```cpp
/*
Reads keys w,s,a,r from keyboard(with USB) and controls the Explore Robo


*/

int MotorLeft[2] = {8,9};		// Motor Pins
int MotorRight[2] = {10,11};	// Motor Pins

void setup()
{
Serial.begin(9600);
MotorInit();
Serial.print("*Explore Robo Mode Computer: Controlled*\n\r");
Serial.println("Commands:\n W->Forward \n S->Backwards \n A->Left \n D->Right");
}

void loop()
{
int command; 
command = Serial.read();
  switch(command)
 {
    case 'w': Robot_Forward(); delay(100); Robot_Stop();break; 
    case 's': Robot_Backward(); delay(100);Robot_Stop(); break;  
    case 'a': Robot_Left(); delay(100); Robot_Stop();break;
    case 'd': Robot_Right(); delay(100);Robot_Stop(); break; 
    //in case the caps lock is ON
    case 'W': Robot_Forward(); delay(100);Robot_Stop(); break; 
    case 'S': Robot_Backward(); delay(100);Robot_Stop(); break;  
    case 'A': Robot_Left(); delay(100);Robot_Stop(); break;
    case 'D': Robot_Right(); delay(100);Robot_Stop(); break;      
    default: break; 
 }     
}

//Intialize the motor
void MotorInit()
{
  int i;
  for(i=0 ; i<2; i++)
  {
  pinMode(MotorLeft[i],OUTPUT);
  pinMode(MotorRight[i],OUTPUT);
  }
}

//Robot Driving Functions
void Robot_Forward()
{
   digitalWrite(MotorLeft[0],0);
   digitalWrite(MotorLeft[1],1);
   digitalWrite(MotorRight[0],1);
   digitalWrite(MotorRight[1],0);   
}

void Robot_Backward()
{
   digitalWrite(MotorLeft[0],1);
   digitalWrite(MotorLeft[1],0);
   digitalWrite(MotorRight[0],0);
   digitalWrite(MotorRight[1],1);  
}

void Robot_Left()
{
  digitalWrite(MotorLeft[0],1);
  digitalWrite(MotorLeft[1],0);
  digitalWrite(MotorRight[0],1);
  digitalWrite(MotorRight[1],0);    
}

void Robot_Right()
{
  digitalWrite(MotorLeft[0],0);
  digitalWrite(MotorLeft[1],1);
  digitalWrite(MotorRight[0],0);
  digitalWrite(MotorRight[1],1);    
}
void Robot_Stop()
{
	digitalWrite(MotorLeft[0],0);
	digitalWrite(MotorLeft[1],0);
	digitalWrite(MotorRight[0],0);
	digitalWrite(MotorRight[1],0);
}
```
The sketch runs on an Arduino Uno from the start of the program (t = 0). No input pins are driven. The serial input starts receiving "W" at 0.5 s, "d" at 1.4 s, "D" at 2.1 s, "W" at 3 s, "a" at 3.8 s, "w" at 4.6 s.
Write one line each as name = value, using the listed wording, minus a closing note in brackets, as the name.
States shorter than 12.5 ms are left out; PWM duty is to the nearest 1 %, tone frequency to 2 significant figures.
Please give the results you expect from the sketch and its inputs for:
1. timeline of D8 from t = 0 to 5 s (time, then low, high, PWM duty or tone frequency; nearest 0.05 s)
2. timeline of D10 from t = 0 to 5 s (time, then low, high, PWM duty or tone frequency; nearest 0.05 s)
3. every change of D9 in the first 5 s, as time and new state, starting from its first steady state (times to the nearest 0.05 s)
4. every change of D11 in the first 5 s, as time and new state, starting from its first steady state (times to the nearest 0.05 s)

timeline of D8 from t = 0 to 5 s = 0 s low; 3.8 s high; 3.9 s low
timeline of D10 from t = 0 to 5 s = 0 s low; 0.5 s high; 0.6 s low; 3 s high; 3.1 s low; 3.8 s high; 3.9 s low; 4.6 s high; 4.7 s low
every change of D9 in the first 5 s, as time and new state, starting from its first steady state = 0 s low; 0.5 s high; 0.6 s low; 1.4 s high; 1.5 s low; 2.1 s high; 2.2 s low; 3 s high; 3.1 s low; 4.6 s high; 4.7 s low
every change of D11 in the first 5 s, as time and new state, starting from its first steady state = 0 s low; 1.4 s high; 1.5 s low; 2.1 s high; 2.2 s low
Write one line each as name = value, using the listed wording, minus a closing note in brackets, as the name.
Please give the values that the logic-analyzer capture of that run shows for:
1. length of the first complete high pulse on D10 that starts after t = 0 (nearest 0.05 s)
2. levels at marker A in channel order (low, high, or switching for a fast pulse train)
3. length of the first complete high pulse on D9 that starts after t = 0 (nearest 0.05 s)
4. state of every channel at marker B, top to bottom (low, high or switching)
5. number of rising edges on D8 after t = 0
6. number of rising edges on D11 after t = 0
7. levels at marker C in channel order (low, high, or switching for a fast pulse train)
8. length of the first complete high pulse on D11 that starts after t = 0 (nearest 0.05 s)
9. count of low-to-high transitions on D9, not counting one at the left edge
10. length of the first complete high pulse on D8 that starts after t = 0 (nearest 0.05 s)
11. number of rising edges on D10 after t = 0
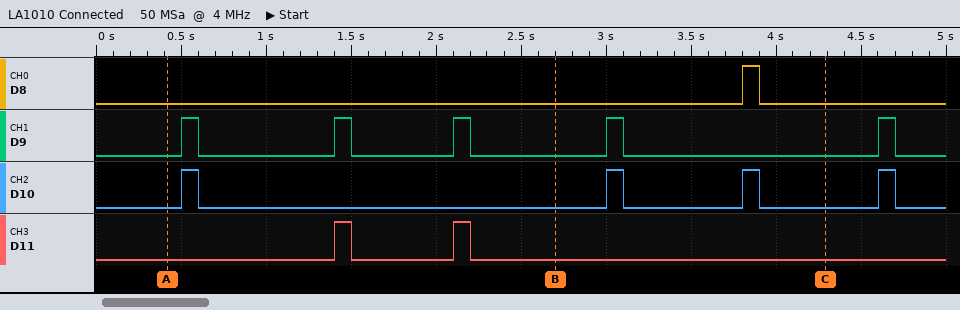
length of the first complete high pulse on D10 that starts after t = 0 = 0.10 s
levels at marker A in channel order = D8 low, D9 low, D10 low, D11 low
length of the first complete high pulse on D9 that starts after t = 0 = 0.10 s
state of every channel at marker B, top to bottom = D8 low, D9 low, D10 low, D11 low
number of rising edges on D8 after t = 0 = 1
number of rising edges on D11 after t = 0 = 2
levels at marker C in channel order = D8 low, D9 low, D10 low, D11 low
length of the first complete high pulse on D11 that starts after t = 0 = 0.10 s
count of low-to-high transitions on D9, not counting one at the left edge = 5
length of the first complete high pulse on D8 that starts after t = 0 = 0.10 s
number of rising edges on D10 after t = 0 = 4
